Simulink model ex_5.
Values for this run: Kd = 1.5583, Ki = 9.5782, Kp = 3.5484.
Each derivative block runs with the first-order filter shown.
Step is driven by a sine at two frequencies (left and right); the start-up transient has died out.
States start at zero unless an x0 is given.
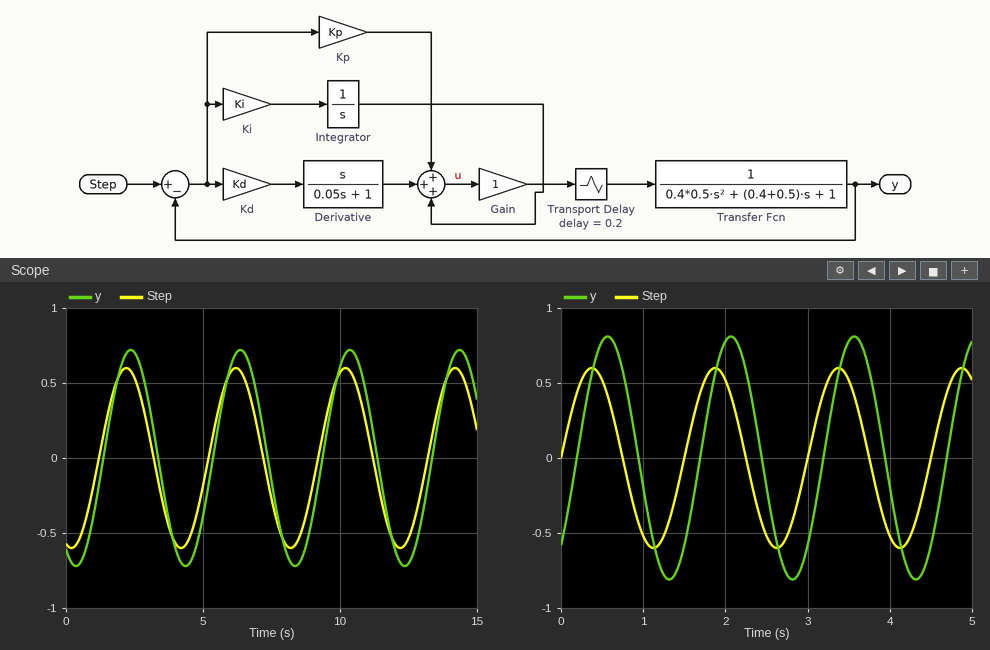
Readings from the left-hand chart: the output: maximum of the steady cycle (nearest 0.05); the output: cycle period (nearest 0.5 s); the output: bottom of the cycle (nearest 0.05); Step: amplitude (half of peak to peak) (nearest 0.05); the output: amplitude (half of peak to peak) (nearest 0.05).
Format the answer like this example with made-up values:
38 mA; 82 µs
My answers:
0.70; 4.0 s; -0.70; 0.60; 0.70
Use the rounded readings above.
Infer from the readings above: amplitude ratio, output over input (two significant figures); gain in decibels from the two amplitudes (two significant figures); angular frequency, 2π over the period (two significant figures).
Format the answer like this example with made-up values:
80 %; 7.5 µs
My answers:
1.2; 1.3 dB; 1.6 rad/s
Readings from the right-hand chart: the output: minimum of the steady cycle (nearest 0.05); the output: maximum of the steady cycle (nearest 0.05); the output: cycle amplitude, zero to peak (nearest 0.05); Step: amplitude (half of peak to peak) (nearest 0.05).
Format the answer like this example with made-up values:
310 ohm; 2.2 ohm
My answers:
-0.80; 0.80; 0.80; 0.60
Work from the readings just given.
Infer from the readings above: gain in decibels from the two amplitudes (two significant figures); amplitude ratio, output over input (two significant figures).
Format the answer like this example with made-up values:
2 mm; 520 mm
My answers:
2.5 dB; 1.3
